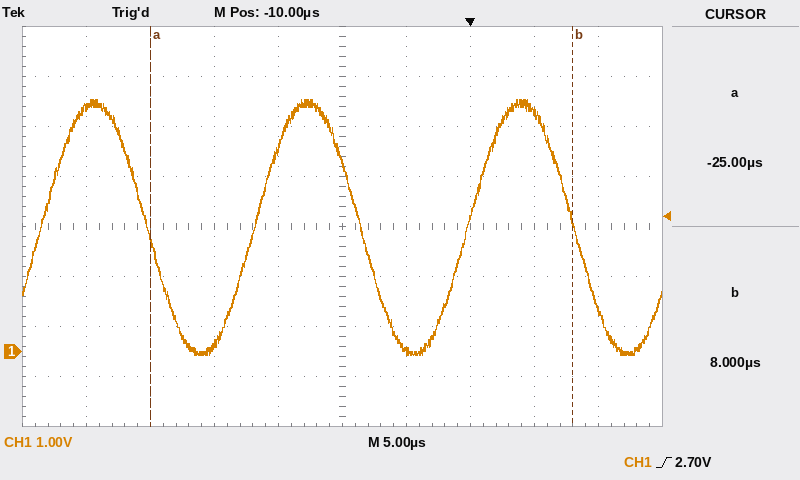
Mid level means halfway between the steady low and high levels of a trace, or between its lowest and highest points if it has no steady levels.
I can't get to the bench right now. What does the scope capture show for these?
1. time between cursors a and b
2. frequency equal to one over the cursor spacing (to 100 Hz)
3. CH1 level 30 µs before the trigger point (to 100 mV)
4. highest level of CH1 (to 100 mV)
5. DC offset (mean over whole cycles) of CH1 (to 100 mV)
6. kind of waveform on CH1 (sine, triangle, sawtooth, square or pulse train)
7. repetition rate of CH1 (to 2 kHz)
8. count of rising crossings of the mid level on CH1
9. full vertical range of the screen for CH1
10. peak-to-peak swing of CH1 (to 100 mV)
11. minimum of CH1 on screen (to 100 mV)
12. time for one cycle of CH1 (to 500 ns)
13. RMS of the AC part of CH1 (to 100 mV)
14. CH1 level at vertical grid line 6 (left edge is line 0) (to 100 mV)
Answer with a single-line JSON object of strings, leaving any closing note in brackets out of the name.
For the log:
{"time between cursors a and b": "33.0 µs", "frequency equal to one over the cursor spacing": "30.3 kHz", "CH1 level 30 µs before the trigger point": "4.9 V", "highest level of CH1": "5.0 V", "DC offset (mean over whole cycles) of CH1": "2.5 V", "kind of waveform on CH1": "sine", "repetition rate of CH1": "60 kHz", "count of rising crossings of the mid level on CH1": "3", "full vertical range of the screen for CH1": "8 V", "peak-to-peak swing of CH1": "5.1 V", "minimum of CH1 on screen": "-100 mV", "time for one cycle of CH1": "16.5 µs", "RMS of the AC part of CH1": "1.8 V", "CH1 level at vertical grid line 6 (left edge is line 0)": "0.0 V"}
